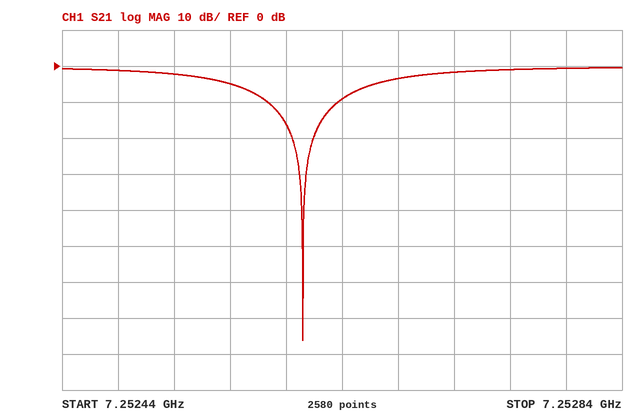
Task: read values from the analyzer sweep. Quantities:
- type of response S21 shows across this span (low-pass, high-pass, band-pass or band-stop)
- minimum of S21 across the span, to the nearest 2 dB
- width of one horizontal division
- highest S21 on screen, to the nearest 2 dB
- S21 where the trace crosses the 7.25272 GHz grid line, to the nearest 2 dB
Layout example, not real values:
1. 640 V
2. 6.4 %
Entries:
1. band-stop
2. -76 dB
3. 40 kHz
4. 0 dB
5. -2 dB
